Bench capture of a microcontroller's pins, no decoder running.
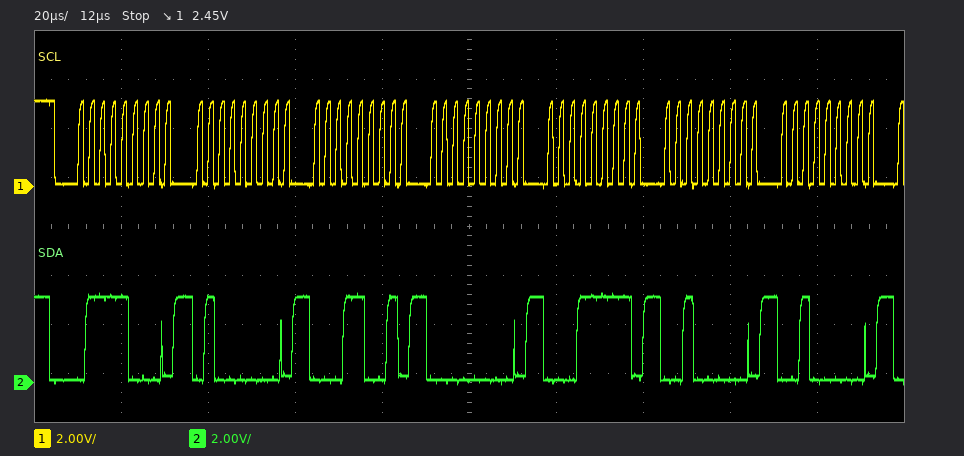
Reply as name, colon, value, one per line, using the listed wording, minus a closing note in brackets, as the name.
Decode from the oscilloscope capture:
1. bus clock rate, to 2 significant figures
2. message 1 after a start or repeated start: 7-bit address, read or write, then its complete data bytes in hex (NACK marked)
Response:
bus clock rate, to 2 significant figures: 400 kHz
message 1 after a start or repeated start: 7-bit address, read or write, then its complete data bytes in hex: 0x3C write: 40 19 00 1F 20 20
